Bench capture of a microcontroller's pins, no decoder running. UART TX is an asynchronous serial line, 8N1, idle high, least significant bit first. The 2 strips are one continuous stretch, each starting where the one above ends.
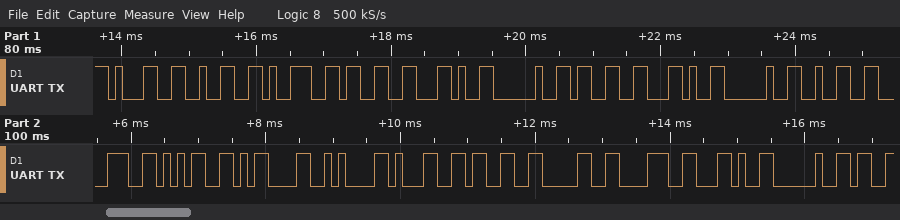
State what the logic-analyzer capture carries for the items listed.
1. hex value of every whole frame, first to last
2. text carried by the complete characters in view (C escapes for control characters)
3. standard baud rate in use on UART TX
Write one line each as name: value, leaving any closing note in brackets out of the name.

hex value of every whole frame, first to last: 31 32 39 33 2C 20 33 2C 20 32 38 35 0D 0A 31 33 30 38 2C 20
text carried by the complete characters in view: "1293, 3, 285\r\n1308, "
standard baud rate in use on UART TX: 9600 baud
